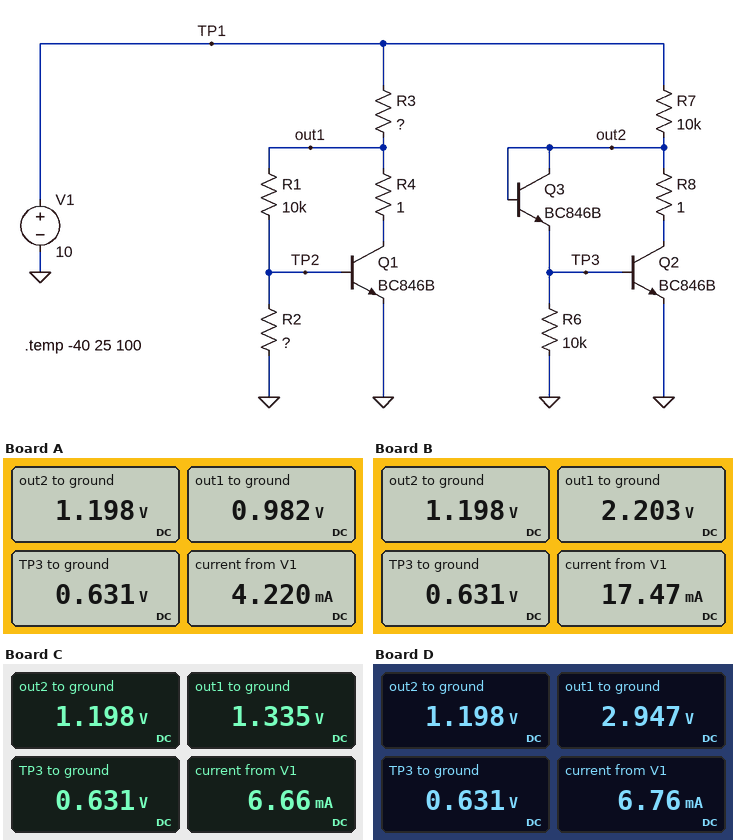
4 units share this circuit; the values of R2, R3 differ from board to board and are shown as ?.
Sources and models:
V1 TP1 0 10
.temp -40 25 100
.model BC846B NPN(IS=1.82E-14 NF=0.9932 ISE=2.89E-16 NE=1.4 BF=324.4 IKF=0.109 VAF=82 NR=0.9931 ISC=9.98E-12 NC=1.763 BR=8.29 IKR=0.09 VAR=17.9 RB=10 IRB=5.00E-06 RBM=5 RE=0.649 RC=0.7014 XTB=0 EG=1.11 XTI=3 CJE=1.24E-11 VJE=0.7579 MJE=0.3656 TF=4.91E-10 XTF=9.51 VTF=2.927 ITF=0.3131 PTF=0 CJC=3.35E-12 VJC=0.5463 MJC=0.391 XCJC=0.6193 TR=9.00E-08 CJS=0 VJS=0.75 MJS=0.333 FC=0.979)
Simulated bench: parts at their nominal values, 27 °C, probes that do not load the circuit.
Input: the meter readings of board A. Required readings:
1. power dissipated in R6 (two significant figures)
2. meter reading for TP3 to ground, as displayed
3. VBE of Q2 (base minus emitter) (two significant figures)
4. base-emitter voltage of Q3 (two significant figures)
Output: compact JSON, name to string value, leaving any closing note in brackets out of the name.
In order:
{"power dissipated in R6": "40 µW", "meter reading for TP3 to ground, as displayed": "0.631 V", "VBE of Q2 (base minus emitter)": "630 mV", "base-emitter voltage of Q3": "570 mV"}
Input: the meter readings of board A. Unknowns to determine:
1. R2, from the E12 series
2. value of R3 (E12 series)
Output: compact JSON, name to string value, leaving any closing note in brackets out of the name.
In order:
{"R2, from the E12 series": "33 kΩ", "value of R3": "2.7 kΩ"}
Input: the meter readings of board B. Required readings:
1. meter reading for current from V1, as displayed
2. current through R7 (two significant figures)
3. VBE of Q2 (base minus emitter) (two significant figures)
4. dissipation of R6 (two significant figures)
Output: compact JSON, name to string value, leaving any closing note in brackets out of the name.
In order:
{"meter reading for current from V1, as displayed": "17.47 mA", "current through R7": "880 µA", "VBE of Q2 (base minus emitter)": "630 mV", "dissipation of R6": "40 µW"}
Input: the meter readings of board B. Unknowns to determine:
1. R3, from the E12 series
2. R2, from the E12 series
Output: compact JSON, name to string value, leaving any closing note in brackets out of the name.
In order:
{"R3, from the E12 series": "470 Ω", "R2, from the E12 series": "8.2 kΩ"}
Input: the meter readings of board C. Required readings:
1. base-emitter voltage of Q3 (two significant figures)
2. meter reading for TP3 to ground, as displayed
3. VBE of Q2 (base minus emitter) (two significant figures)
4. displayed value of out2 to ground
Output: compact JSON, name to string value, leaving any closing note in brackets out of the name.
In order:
{"base-emitter voltage of Q3": "570 mV", "meter reading for TP3 to ground, as displayed": "0.631 V", "VBE of Q2 (base minus emitter)": "630 mV", "displayed value of out2 to ground": "1.198 V"}
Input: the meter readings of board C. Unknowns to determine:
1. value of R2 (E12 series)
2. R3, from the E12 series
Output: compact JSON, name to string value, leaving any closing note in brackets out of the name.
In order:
{"value of R2": "15 kΩ", "R3, from the E12 series": "1.5 kΩ"}
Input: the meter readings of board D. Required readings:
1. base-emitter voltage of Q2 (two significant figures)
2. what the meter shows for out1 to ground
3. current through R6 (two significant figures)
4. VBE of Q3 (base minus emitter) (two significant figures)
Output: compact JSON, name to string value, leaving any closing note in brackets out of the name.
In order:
{"base-emitter voltage of Q2": "630 mV", "what the meter shows for out1 to ground": "2.947 V", "current through R6": "63 µA", "VBE of Q3 (base minus emitter)": "570 mV"}
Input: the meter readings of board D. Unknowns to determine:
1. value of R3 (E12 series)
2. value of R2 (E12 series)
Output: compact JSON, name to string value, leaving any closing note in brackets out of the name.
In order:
{"value of R3": "1.2 kΩ", "value of R2": "3.3 kΩ"}
